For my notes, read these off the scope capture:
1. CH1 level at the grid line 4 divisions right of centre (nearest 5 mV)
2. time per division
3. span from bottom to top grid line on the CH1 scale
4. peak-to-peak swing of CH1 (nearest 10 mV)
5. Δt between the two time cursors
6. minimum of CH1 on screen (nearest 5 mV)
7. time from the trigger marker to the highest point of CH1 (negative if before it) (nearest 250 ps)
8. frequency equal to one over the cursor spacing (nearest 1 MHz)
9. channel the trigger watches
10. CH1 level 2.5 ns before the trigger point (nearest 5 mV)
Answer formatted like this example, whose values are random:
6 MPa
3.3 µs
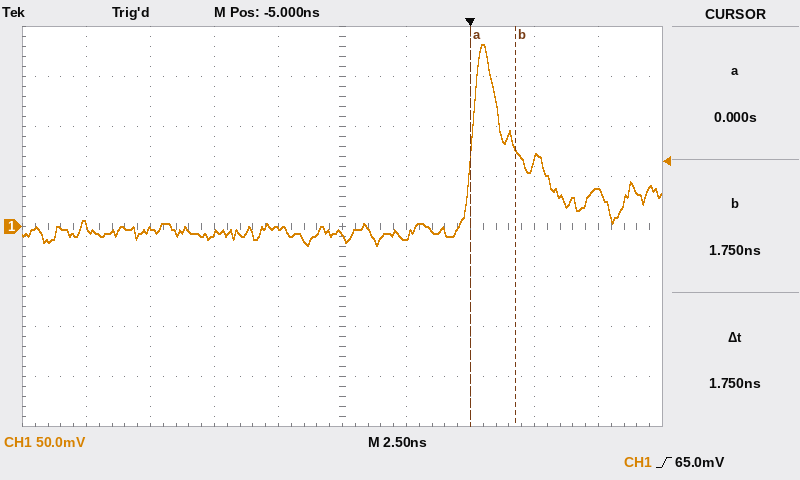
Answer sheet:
35 mV
2.5 ns
400 mV
200 mV
1.75 ns
-20 mV
+500 ps
571 MHz
CH1
-10 mV
